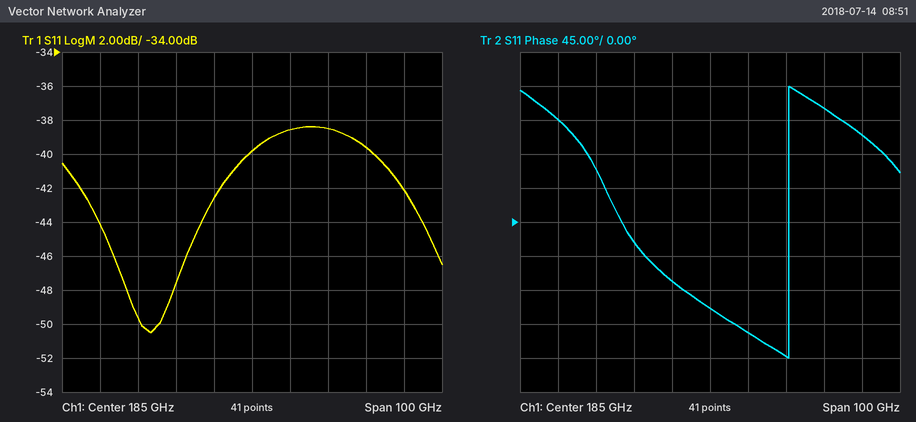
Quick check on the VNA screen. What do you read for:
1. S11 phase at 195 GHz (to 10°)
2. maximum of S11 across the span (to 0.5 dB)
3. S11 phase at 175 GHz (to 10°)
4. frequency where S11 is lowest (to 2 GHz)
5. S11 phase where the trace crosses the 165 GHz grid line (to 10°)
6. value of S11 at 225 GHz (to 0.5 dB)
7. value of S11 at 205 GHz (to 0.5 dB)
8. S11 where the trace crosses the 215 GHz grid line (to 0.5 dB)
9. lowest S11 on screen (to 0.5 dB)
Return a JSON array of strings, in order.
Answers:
["-150°", "-38.5 dB", "-80°", "158 GHz", "-30°", "-42.0 dB", "-38.5 dB", "-39.5 dB", "-50.5 dB"]
